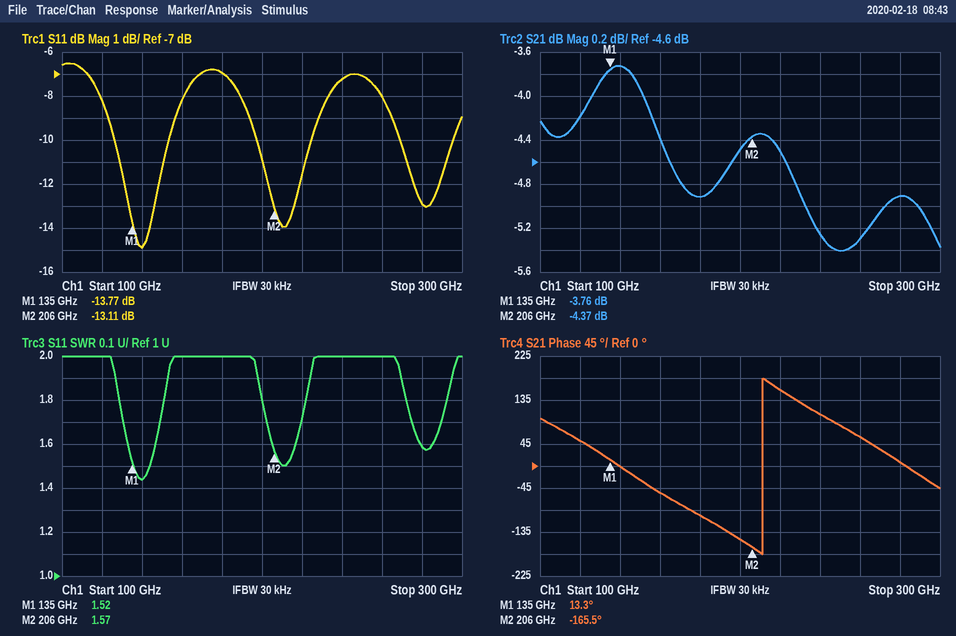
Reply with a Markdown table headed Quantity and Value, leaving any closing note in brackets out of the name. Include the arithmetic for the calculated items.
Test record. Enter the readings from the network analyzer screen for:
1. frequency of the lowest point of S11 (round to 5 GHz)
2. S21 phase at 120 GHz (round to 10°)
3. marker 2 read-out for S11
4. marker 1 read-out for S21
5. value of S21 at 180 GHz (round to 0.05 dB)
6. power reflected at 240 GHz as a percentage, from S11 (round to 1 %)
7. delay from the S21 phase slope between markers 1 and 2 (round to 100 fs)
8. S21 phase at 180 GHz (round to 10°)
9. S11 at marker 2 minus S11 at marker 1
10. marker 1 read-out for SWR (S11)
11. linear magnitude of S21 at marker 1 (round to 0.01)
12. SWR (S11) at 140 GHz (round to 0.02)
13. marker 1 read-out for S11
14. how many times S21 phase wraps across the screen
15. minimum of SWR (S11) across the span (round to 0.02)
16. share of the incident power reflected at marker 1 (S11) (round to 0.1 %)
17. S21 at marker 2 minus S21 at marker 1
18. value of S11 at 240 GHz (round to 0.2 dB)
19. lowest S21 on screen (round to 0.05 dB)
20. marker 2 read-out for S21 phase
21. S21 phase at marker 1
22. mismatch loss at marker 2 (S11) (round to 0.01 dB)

| Quantity | Value |
|---|---|
| frequency of the lowest point of S11 | 140 GHz |
| S21 phase at 120 GHz | 50° |
| marker 2 read-out for S11 | -13.11 dB |
| marker 1 read-out for S21 | -3.76 dB |
| value of S21 at 180 GHz | -4.90 dB |
| power reflected at 240 GHz as a percentage, from S11 | 10^(-7.2/10) ≈ 19 % |
| delay from the S21 phase slope between markers 1 and 2 | −(-165.5° − (13.3°))/(360° × 71 GHz) ≈ 7.0 ps |
| S21 phase at 180 GHz | -100° |
| S11 at marker 2 minus S11 at marker 1 | -13.11 − (-13.77) = 0.66 dB |
| marker 1 read-out for SWR | 1.52 |
| linear magnitude of S21 at marker 1 | 10^(-3.76/20) ≈ 0.65 |
| SWR (S11) at 140 GHz | 1.44 |
| marker 1 read-out for S11 | -13.77 dB |
| how many times S21 phase wraps across the screen | 1 |
| minimum of SWR (S11) across the span | 1.44 |
| share of the incident power reflected at marker 1 (S11) | 10^(-13.77/10) ≈ 4.2 % |
| S21 at marker 2 minus S21 at marker 1 | -4.37 − (-3.76) = -0.61 dB |
| value of S11 at 240 GHz | -7.2 dB |
| lowest S21 on screen | -5.40 dB |
| marker 2 read-out for S21 phase | -165.5° |
| S21 phase at marker 1 | 13.3° |
| mismatch loss at marker 2 (S11) | −10 log10(1 − 10^(-13.11/10)) ≈ 0.22 dB |
